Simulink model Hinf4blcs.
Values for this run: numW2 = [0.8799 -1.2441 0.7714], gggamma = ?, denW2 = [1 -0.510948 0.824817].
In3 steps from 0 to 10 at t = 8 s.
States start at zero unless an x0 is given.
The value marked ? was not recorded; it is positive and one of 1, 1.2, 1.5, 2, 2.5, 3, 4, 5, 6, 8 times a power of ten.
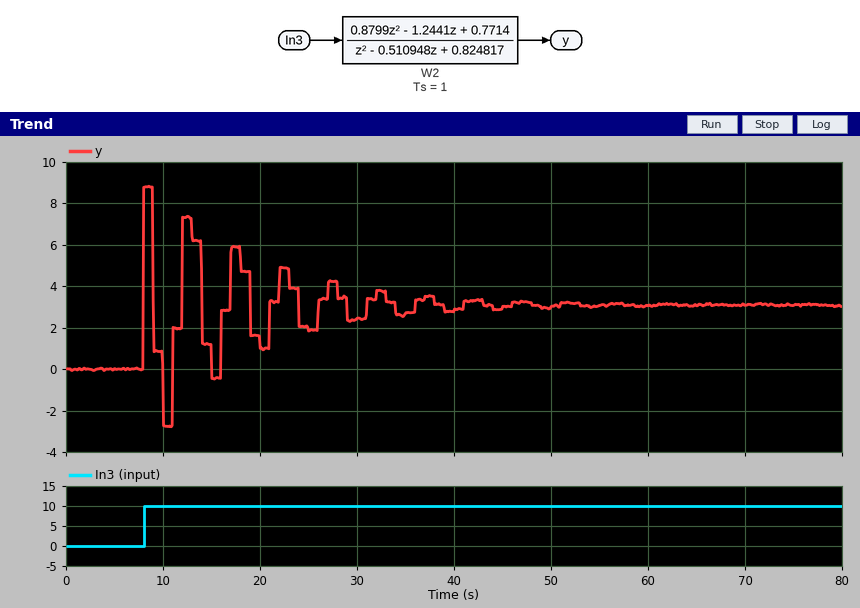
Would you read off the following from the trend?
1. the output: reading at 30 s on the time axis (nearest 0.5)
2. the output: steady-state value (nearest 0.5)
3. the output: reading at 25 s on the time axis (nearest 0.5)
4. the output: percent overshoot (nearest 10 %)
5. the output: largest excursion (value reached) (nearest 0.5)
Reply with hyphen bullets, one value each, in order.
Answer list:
- 2.5
- 3.0
- 2.0
- 180 %
- 9.0
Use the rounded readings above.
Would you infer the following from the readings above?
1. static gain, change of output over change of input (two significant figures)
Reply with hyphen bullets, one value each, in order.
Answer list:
- 0.30
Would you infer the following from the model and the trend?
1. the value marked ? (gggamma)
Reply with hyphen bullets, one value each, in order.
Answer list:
- 1
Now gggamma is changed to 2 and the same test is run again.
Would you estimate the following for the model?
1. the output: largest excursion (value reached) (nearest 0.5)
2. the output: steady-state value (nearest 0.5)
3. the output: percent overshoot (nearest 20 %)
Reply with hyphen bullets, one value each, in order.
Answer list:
- 4.5
- 1.5
- 180 %
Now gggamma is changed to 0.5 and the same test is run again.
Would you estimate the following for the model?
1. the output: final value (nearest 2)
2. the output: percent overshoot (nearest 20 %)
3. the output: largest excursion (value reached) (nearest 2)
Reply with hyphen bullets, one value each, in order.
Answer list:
- 6
- 180 %
- 18
